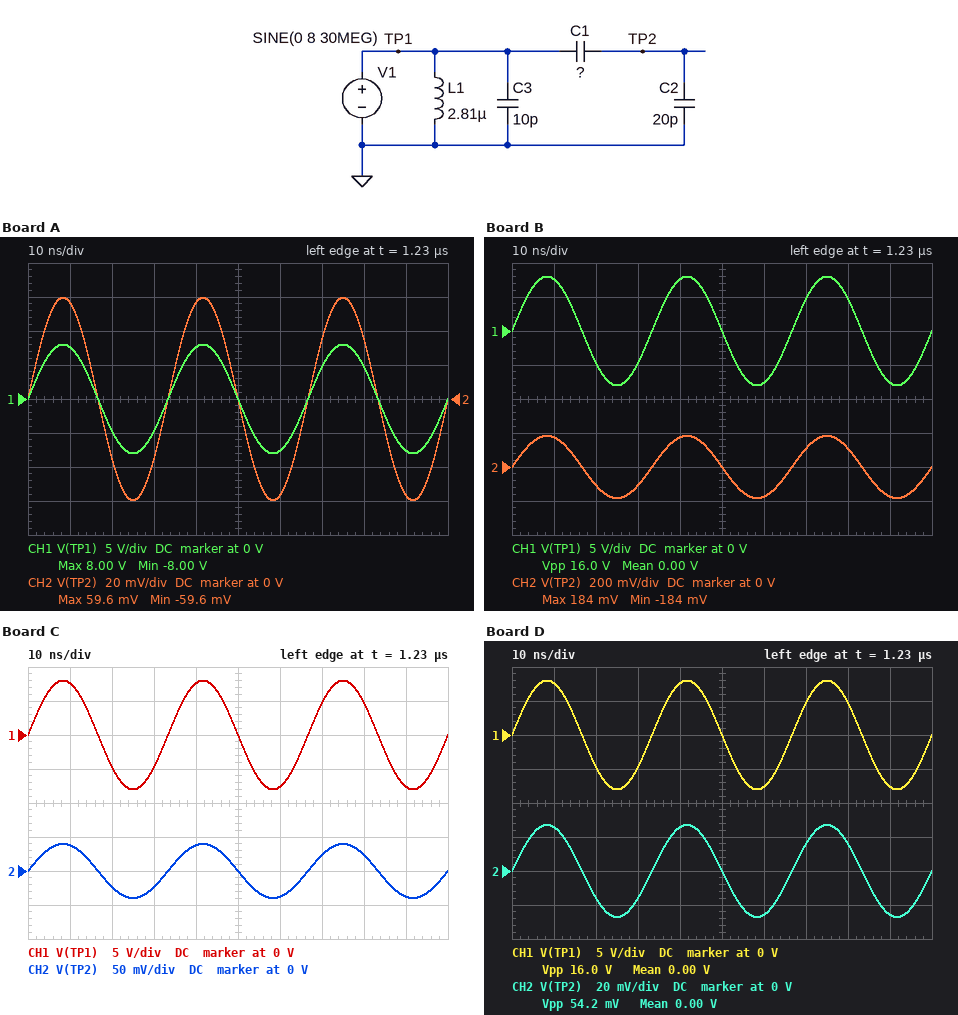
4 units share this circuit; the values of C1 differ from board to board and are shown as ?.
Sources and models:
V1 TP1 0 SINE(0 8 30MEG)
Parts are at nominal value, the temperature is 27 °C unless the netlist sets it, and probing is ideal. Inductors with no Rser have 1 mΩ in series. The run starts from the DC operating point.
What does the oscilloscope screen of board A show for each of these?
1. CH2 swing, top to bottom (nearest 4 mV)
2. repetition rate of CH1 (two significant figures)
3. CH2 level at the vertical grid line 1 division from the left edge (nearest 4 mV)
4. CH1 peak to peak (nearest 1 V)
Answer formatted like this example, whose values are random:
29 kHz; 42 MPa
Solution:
120 mV; 30 MHz; 56 mV; 16 V
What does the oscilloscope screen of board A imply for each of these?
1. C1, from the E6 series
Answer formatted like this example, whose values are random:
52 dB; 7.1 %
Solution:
150 fF
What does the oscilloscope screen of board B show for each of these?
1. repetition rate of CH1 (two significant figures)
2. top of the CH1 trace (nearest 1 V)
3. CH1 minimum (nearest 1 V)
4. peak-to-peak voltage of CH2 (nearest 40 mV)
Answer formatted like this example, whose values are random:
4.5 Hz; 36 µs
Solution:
30 MHz; 8 V; -8 V; 360 mV
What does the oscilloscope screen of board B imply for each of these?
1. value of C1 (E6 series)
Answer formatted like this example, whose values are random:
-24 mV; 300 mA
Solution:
470 fF
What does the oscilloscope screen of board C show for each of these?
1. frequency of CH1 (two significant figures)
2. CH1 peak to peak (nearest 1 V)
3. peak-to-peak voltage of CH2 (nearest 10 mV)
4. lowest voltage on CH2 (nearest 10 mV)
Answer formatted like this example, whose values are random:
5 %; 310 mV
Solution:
30 MHz; 16 V; 80 mV; -40 mV
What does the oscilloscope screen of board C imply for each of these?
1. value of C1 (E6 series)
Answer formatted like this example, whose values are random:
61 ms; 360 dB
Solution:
100 fF
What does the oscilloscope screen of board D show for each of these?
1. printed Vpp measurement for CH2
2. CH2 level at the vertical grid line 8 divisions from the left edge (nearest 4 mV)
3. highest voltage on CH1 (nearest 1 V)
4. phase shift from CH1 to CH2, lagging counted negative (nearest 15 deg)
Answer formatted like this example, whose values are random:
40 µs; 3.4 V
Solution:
54.2 mV; 16 mV; 8 V; 0 deg
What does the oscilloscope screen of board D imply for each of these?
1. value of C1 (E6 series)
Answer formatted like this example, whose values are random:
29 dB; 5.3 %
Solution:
68 fF
